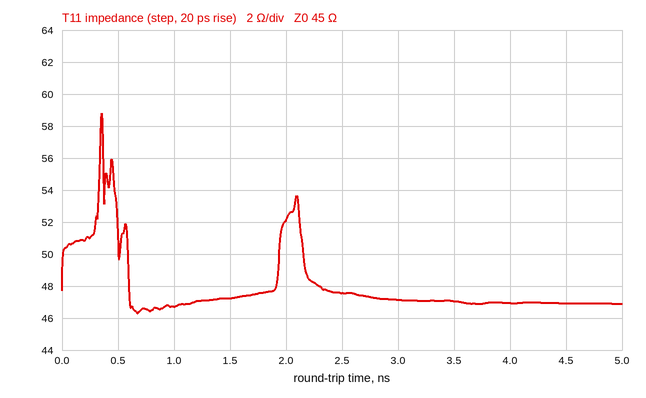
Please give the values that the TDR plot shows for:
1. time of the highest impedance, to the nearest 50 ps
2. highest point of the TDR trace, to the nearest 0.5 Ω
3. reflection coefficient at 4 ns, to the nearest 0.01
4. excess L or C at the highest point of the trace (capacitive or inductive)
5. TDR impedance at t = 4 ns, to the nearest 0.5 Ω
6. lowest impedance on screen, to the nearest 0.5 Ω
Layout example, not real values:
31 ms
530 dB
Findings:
350 ps
59.0 Ω
+0.02
inductive
47.0 Ω
46.5 Ω
